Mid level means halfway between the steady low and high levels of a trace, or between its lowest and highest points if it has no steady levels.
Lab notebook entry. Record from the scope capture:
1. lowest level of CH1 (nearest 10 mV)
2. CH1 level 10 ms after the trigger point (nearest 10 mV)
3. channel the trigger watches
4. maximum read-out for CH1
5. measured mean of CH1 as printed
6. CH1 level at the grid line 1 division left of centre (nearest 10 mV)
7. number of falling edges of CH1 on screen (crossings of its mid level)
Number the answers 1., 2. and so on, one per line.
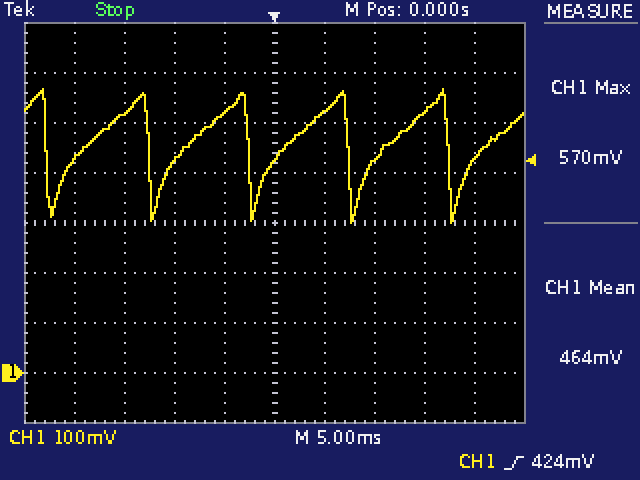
1. 300 mV
2. 420 mV
3. CH1
4. 570 mV
5. 464 mV
6. 520 mV
7. 5
